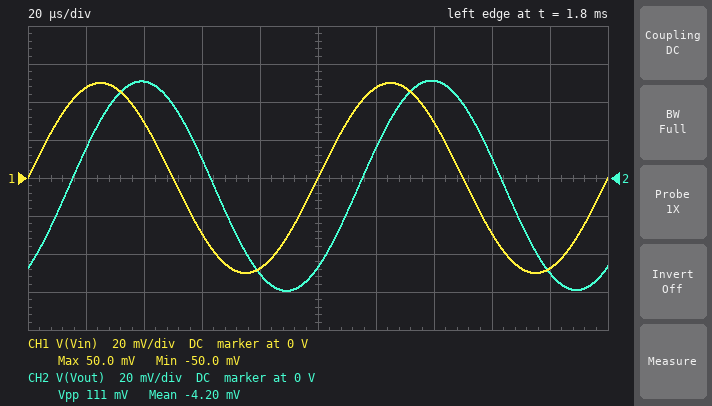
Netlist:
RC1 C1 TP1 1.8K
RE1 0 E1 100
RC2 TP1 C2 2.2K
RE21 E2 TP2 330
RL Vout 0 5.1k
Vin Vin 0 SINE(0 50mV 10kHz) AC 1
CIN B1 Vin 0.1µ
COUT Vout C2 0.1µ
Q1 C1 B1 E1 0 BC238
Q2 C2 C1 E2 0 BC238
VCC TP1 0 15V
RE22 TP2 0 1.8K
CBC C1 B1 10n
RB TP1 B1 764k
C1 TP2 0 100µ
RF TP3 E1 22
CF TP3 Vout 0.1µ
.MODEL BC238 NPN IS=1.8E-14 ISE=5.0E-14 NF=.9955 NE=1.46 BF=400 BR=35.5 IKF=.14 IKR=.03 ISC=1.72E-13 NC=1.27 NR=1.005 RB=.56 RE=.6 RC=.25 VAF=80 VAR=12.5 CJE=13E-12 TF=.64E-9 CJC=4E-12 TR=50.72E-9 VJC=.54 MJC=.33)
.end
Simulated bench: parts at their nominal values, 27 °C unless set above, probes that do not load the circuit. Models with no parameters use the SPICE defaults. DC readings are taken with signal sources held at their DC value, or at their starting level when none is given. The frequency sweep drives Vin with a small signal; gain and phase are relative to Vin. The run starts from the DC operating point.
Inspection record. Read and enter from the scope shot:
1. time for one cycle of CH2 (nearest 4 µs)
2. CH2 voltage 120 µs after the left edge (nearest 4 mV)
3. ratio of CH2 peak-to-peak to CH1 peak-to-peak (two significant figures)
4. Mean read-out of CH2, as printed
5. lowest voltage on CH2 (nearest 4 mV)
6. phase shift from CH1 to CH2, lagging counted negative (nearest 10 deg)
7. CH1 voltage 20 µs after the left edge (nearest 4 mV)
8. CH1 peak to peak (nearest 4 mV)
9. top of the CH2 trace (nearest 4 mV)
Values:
100 µs
16 mV
1.1
-4.20 mV
-60 mV
-50 deg
48 mV
100 mV
52 mV
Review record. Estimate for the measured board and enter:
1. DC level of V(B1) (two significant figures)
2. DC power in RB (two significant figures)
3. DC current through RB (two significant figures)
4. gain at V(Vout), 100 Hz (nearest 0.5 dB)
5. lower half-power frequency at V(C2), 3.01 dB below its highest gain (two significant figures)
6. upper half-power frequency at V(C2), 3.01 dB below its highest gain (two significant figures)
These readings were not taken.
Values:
1.2 V
250 µW
18 µA
20.5 dB
22 Hz
530 Hz
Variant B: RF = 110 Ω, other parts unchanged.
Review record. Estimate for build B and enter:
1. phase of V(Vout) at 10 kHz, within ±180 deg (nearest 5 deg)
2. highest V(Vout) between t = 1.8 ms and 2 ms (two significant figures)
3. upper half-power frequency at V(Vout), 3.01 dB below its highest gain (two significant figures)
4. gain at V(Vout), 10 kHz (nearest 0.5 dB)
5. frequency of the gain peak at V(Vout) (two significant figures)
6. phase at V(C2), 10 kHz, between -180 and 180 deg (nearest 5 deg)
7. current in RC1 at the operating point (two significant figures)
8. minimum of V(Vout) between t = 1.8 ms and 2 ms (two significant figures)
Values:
-40 deg
70 mV
680 Hz
3.5 dB
270 Hz
-60 deg
5.5 mA
-78 mV
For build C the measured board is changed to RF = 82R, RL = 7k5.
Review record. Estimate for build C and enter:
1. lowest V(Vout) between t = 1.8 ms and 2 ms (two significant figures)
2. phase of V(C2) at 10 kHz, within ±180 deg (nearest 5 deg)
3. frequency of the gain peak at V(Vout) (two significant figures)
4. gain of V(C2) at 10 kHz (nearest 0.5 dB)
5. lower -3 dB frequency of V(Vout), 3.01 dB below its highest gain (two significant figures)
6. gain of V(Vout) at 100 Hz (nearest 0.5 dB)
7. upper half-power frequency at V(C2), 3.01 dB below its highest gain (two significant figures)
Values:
-73 mV
-65 deg
230 Hz
6.0 dB
85 Hz
22.5 dB
510 Hz
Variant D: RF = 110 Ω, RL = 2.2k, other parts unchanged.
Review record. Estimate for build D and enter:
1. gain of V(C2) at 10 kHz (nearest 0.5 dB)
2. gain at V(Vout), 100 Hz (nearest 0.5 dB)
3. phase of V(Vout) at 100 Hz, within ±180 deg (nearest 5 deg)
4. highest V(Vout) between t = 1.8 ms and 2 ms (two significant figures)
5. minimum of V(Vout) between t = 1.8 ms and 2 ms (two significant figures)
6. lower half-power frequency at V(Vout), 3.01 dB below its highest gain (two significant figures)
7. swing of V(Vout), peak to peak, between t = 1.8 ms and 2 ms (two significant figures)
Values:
6.5 dB
14.0 dB
80 deg
72 mV
-74 mV
190 Hz
150 mV
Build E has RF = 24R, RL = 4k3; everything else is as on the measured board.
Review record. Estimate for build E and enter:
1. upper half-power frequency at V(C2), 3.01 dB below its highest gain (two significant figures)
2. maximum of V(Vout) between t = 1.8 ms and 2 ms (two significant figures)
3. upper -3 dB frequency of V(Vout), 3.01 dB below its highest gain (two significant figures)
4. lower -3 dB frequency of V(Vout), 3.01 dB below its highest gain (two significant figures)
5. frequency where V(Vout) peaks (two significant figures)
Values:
540 Hz
52 mV
720 Hz
130 Hz
300 Hz
